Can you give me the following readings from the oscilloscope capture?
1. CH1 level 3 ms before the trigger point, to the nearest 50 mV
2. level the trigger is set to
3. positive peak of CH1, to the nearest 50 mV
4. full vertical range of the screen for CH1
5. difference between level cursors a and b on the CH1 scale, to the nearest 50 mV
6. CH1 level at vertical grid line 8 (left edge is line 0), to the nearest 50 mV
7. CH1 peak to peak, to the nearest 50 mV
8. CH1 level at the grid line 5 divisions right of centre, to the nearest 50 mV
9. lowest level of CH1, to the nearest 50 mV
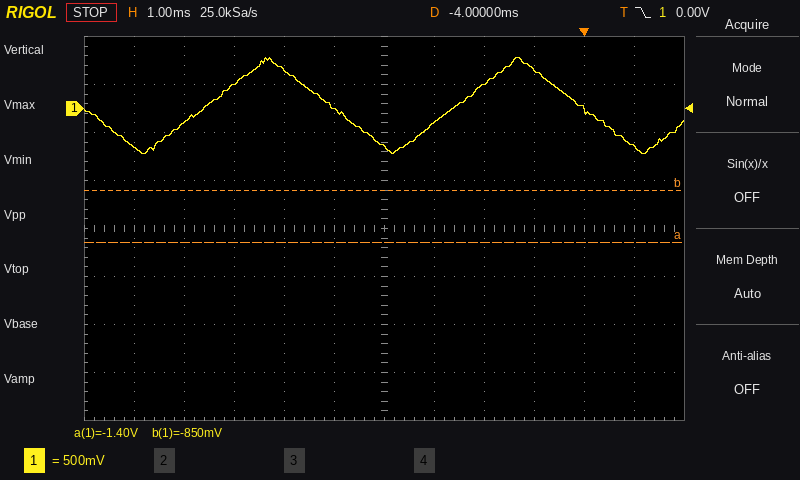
-150 mV
0.00 V
550 mV
4 V
550 mV
250 mV
1.00 V
-400 mV
-450 mV
